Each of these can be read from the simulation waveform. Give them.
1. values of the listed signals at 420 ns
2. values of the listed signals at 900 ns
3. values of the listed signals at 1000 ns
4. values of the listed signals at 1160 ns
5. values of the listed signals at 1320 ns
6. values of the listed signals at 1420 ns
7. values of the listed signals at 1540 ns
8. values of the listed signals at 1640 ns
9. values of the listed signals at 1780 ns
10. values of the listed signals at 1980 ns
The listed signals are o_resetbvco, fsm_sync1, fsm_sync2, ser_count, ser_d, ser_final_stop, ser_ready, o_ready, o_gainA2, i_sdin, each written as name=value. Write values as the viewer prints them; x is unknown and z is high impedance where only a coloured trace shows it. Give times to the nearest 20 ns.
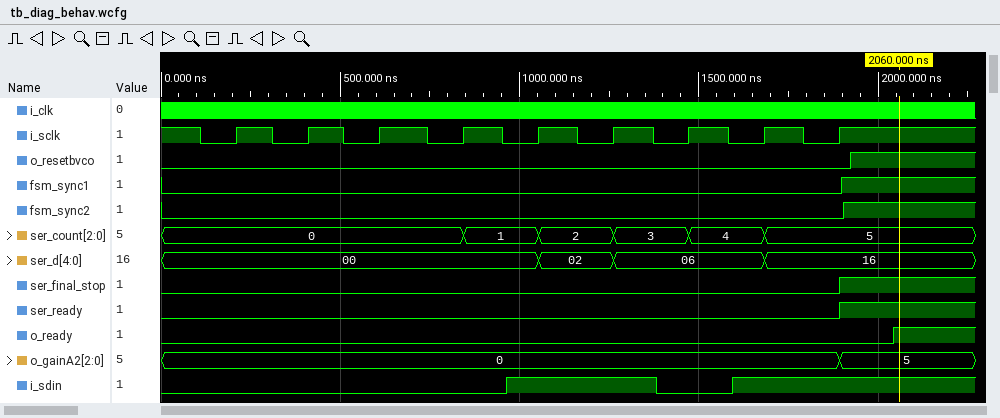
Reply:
o_resetbvco=0, fsm_sync1=0, fsm_sync2=0, ser_count=0, ser_d=00, ser_final_stop=0, ser_ready=0, o_ready=0, o_gainA2=0, i_sdin=0
o_resetbvco=0, fsm_sync1=0, fsm_sync2=0, ser_count=1, ser_d=00, ser_final_stop=0, ser_ready=0, o_ready=0, o_gainA2=0, i_sdin=0
o_resetbvco=0, fsm_sync1=0, fsm_sync2=0, ser_count=1, ser_d=00, ser_final_stop=0, ser_ready=0, o_ready=0, o_gainA2=0, i_sdin=1
o_resetbvco=0, fsm_sync1=0, fsm_sync2=0, ser_count=2, ser_d=02, ser_final_stop=0, ser_ready=0, o_ready=0, o_gainA2=0, i_sdin=1
o_resetbvco=0, fsm_sync1=0, fsm_sync2=0, ser_count=3, ser_d=06, ser_final_stop=0, ser_ready=0, o_ready=0, o_gainA2=0, i_sdin=1
o_resetbvco=0, fsm_sync1=0, fsm_sync2=0, ser_count=3, ser_d=06, ser_final_stop=0, ser_ready=0, o_ready=0, o_gainA2=0, i_sdin=0
o_resetbvco=0, fsm_sync1=0, fsm_sync2=0, ser_count=4, ser_d=06, ser_final_stop=0, ser_ready=0, o_ready=0, o_gainA2=0, i_sdin=0
o_resetbvco=0, fsm_sync1=0, fsm_sync2=0, ser_count=4, ser_d=06, ser_final_stop=0, ser_ready=0, o_ready=0, o_gainA2=0, i_sdin=1
o_resetbvco=0, fsm_sync1=0, fsm_sync2=0, ser_count=5, ser_d=16, ser_final_stop=0, ser_ready=0, o_ready=0, o_gainA2=0, i_sdin=1
o_resetbvco=1, fsm_sync1=1, fsm_sync2=1, ser_count=5, ser_d=16, ser_final_stop=1, ser_ready=1, o_ready=0, o_gainA2=5, i_sdin=1
